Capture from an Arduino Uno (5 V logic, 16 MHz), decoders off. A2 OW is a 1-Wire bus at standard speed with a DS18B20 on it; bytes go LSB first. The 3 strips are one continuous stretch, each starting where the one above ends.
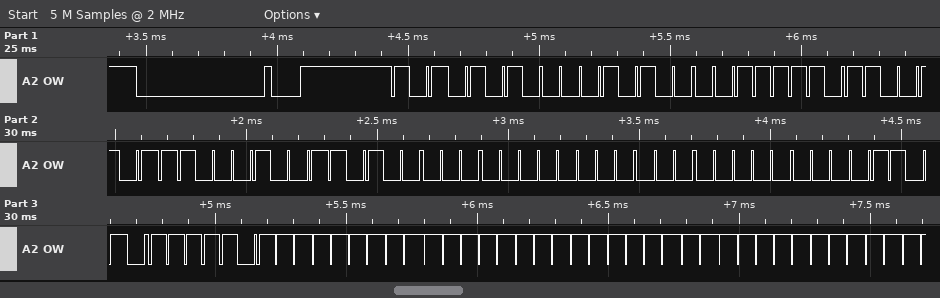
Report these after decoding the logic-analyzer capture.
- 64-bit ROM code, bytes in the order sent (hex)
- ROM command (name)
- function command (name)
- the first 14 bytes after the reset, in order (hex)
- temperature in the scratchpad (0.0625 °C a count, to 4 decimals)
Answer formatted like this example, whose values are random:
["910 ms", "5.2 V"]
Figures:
["28 7C D3 91 05 00 00 B0", "Match ROM", "Read Scratchpad", "55 28 7C D3 91 05 00 00 B0 BE FF FF FF FF", "-0.0625 °C"]
